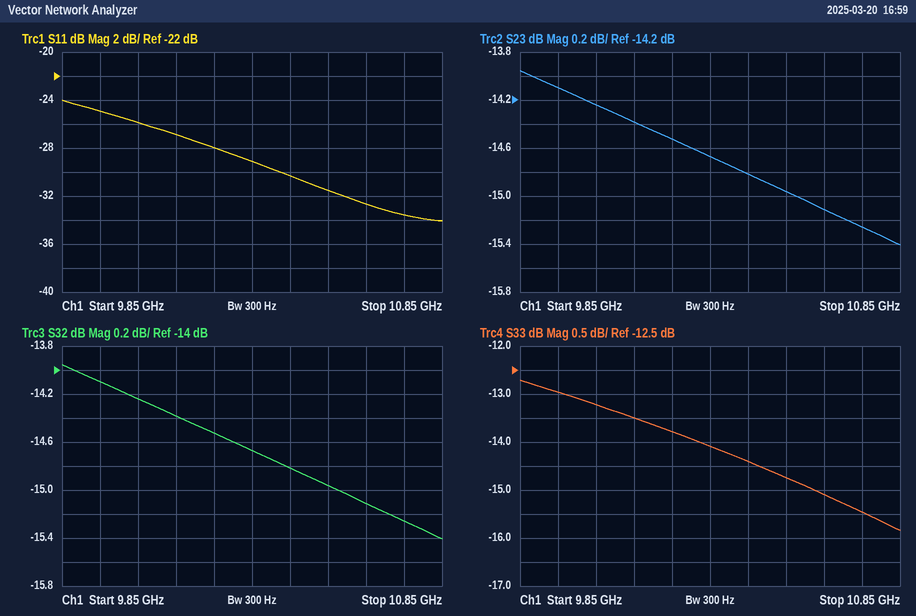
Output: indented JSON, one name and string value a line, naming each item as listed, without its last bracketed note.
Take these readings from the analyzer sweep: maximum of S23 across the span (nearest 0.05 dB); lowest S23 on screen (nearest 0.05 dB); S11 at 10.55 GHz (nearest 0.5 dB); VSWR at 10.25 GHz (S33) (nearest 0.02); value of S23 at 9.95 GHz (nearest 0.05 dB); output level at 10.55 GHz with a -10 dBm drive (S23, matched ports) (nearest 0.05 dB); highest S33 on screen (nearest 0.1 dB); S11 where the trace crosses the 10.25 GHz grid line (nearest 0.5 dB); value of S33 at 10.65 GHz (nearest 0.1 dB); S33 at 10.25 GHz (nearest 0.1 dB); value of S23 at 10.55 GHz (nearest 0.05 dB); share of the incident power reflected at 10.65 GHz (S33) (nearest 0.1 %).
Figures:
{
  "maximum of S23 across the span": "-13.95 dB",
  "lowest S23 on screen": "-15.40 dB",
  "S11 at 10.55 GHz": "-31.5 dB",
  "VSWR at 10.25 GHz (S33)": "1.52",
  "value of S23 at 9.95 GHz": "-14.10 dB",
  "output level at 10.55 GHz with a -10 dBm drive (S23, matched ports)": "-24.95 dBm",
  "highest S33 on screen": "-12.7 dB",
  "S11 where the trace crosses the 10.25 GHz grid line": "-28.0 dB",
  "value of S33 at 10.65 GHz": "-15.1 dB",
  "S33 at 10.25 GHz": "-13.8 dB",
  "value of S23 at 10.55 GHz": "-14.95 dB",
  "share of the incident power reflected at 10.65 GHz (S33)": "3.1 %"
}
